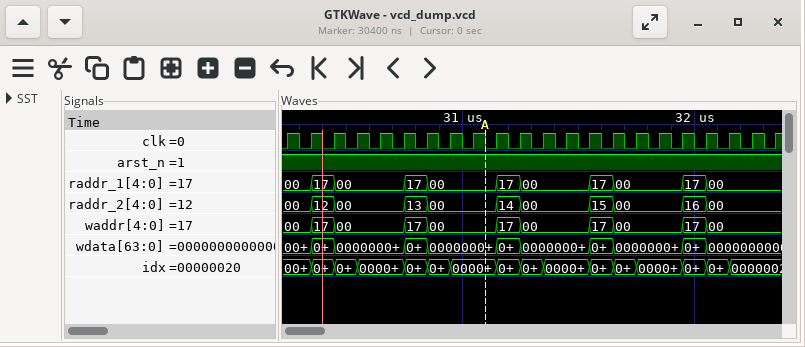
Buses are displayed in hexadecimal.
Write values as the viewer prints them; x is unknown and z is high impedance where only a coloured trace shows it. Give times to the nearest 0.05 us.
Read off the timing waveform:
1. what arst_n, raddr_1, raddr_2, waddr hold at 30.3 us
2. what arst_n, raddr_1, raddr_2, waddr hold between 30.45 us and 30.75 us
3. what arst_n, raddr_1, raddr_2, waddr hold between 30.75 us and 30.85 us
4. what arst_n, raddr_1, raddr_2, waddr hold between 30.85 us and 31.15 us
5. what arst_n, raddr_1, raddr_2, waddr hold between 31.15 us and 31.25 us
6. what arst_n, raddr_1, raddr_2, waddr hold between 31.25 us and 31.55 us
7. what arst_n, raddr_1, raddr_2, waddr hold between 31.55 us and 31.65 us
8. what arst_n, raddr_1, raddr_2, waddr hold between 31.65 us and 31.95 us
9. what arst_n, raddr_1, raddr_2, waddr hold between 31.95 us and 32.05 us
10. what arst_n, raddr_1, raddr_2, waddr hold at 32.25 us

arst_n=1, raddr_1=00, raddr_2=00, waddr=00
arst_n=1, raddr_1=00, raddr_2=00, waddr=00
arst_n=1, raddr_1=17, raddr_2=13, waddr=17
arst_n=1, raddr_1=00, raddr_2=00, waddr=00
arst_n=1, raddr_1=17, raddr_2=14, waddr=17
arst_n=1, raddr_1=00, raddr_2=00, waddr=00
arst_n=1, raddr_1=17, raddr_2=15, waddr=17
arst_n=1, raddr_1=00, raddr_2=00, waddr=00
arst_n=1, raddr_1=17, raddr_2=16, waddr=17
arst_n=1, raddr_1=00, raddr_2=00, waddr=00
